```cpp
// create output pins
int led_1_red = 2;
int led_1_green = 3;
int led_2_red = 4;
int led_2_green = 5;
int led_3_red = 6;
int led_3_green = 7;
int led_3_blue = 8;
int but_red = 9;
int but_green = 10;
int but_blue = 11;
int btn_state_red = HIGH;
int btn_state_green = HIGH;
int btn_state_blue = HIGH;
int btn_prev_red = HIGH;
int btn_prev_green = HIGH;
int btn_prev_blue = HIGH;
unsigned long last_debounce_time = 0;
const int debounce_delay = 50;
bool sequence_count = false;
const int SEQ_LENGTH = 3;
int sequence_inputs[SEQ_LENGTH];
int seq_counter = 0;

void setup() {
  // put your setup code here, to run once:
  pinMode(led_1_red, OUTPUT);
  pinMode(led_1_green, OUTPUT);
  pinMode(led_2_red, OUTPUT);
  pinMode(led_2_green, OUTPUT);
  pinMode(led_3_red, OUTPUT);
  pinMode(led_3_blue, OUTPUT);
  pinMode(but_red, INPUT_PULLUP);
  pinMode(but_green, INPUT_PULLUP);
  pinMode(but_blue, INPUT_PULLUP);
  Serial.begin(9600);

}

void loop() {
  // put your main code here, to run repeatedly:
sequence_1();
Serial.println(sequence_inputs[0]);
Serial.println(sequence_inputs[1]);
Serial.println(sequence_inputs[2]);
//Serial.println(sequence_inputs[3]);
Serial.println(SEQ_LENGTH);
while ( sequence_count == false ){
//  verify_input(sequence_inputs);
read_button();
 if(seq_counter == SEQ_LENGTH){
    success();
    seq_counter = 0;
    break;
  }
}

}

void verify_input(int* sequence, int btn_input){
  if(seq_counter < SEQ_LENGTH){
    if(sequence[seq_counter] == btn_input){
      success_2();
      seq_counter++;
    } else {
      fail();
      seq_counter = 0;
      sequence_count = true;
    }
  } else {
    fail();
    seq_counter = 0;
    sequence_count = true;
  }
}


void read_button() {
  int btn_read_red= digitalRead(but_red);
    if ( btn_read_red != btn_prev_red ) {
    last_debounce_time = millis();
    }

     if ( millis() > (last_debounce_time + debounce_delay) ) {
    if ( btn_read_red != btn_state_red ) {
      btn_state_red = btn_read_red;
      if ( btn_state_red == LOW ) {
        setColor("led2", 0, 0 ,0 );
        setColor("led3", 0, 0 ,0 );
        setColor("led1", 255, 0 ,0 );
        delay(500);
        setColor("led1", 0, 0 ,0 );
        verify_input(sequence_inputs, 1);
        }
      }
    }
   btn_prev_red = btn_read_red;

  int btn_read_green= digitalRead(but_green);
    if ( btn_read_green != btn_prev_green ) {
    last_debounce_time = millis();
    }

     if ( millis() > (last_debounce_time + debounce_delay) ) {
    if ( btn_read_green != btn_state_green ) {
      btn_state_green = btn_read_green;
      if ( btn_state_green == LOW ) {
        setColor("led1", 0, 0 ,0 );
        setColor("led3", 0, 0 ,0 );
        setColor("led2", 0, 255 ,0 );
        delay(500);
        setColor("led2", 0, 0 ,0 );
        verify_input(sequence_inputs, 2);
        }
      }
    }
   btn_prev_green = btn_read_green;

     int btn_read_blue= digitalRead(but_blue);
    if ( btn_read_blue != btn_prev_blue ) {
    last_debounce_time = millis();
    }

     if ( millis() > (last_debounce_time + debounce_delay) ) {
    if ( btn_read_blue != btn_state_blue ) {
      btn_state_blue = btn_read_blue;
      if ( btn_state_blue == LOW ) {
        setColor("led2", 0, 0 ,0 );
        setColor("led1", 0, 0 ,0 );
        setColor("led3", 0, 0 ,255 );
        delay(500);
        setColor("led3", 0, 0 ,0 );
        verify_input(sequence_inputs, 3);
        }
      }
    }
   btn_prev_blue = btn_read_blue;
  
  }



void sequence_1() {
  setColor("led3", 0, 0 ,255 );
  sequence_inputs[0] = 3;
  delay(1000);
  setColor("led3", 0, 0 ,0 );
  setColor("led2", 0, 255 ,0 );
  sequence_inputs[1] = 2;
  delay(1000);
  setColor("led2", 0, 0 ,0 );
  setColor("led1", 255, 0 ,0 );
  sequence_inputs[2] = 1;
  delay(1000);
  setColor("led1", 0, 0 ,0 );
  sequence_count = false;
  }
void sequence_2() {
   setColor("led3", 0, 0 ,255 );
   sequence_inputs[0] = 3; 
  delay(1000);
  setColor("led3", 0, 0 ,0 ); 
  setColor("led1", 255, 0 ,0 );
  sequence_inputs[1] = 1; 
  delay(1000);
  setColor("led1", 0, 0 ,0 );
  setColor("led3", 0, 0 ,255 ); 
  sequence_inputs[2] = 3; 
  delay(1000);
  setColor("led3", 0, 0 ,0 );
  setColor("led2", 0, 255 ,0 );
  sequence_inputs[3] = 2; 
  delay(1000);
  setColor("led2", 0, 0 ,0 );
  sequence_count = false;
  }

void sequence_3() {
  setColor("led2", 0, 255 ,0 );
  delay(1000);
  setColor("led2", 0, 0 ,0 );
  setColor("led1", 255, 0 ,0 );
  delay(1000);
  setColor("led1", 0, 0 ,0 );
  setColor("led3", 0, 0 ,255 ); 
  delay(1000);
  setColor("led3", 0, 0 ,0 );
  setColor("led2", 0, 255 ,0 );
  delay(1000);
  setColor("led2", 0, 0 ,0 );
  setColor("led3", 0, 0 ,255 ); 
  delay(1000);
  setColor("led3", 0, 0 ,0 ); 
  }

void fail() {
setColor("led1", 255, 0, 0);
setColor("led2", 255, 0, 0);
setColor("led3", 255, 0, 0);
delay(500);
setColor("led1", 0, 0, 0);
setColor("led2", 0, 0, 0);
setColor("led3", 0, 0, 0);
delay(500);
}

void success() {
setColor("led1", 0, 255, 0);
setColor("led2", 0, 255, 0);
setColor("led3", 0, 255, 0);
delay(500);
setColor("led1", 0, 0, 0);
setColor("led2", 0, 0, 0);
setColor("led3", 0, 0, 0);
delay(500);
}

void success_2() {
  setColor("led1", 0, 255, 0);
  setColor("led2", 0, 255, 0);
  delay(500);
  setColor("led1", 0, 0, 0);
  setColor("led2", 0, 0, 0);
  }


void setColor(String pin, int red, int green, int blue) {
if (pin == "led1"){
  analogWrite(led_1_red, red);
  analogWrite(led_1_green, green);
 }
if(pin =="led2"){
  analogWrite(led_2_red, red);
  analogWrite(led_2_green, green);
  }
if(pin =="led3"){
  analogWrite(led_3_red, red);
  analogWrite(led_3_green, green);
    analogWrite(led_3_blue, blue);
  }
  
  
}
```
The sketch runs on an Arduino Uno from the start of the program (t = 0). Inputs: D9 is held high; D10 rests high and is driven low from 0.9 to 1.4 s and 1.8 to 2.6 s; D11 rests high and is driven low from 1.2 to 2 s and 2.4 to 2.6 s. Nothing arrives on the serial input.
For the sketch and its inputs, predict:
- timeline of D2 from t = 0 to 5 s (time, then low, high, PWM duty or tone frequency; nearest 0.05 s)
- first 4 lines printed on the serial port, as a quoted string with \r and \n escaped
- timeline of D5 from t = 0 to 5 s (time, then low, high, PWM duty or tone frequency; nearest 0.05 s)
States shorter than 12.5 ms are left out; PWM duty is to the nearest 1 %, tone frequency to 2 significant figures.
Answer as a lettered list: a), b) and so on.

a) 0 s low; 2 s high; 3 s low
b) "3\r\n2\r\n1\r\n3\r\n"
c) 0 s low; 1 s high; 2 s low
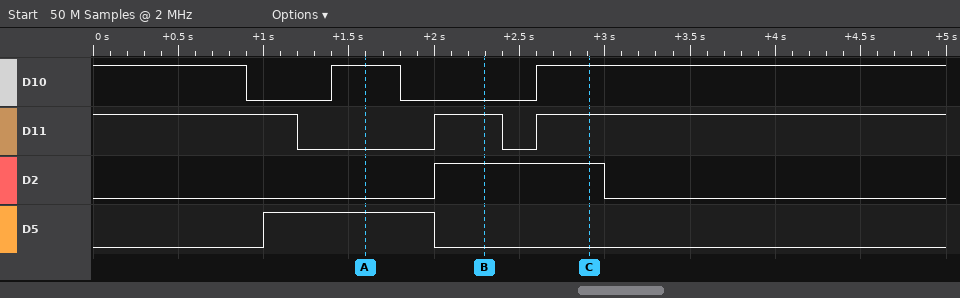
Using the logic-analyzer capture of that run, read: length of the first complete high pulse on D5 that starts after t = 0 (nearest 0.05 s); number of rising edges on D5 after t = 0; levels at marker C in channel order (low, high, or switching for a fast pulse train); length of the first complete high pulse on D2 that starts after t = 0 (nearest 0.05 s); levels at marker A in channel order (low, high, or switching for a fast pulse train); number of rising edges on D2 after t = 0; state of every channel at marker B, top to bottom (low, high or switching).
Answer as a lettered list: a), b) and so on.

a) 1.00 s
b) 1
c) D10 high, D11 high, D2 high, D5 low
d) 1.00 s
e) D10 high, D11 low, D2 low, D5 high
f) 1
g) D10 low, D11 high, D2 high, D5 low
